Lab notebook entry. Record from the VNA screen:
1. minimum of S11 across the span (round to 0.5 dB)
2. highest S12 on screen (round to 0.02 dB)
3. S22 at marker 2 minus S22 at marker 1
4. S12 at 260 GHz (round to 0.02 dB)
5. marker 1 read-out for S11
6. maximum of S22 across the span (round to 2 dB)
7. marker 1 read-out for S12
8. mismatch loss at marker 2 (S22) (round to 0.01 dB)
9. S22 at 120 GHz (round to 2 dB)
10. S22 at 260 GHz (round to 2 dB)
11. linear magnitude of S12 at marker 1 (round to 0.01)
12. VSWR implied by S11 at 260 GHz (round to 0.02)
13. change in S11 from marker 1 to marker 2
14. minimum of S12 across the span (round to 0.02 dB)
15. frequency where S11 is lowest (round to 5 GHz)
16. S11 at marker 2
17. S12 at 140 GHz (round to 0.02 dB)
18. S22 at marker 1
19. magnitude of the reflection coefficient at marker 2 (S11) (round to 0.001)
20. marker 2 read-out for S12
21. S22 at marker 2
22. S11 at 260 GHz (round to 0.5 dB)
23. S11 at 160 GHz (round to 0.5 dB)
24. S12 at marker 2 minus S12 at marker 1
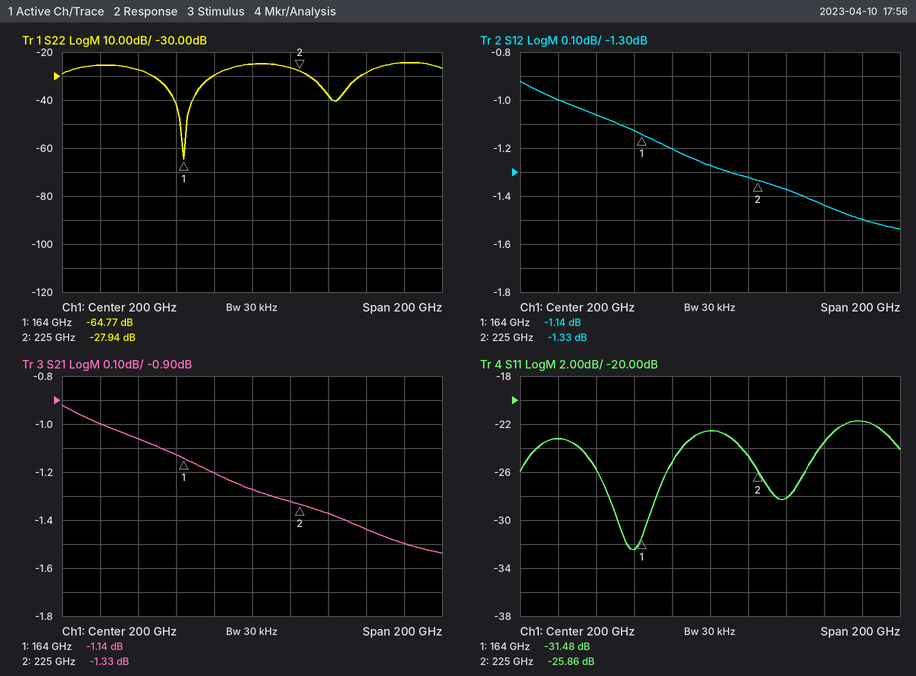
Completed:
-32.5 dB
-0.92 dB
36.83 dB
-1.44 dB
-31.48 dB
-24 dB
-1.14 dB
0.01 dB
-26 dB
-28 dB
0.88
1.14
5.62 dB
-1.54 dB
160 GHz
-25.86 dB
-1.06 dB
-64.77 dB
0.051
-1.33 dB
-27.94 dB
-23.5 dB
-32.5 dB
-0.19 dB
